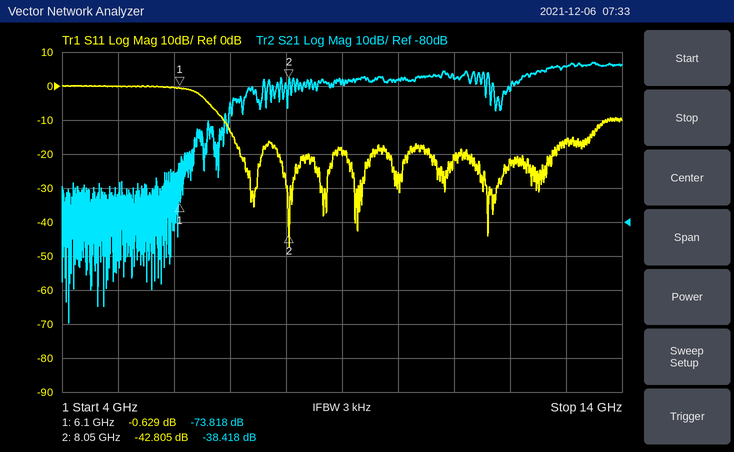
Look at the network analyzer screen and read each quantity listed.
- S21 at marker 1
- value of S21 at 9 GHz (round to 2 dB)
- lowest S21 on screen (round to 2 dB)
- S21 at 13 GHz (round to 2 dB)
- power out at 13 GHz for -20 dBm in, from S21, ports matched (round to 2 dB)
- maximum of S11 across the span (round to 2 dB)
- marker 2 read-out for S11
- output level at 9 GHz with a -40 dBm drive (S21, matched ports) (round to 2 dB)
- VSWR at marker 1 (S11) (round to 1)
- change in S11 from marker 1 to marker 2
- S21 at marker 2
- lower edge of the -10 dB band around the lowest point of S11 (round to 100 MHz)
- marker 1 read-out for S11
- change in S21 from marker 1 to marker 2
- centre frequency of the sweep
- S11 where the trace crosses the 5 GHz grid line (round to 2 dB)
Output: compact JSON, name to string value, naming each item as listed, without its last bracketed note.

{"S21 at marker 1": "-73.818 dB", "value of S21 at 9 GHz": "-38 dB", "lowest S21 on screen": "-110 dB", "S21 at 13 GHz": "-34 dB", "power out at 13 GHz for -20 dBm in, from S21, ports matched": "-54 dBm", "maximum of S11 across the span": "0 dB", "marker 2 read-out for S11": "-42.805 dB", "output level at 9 GHz with a -40 dBm drive (S21, matched ports)": "-78 dBm", "VSWR at marker 1 (S11)": "28", "change in S11 from marker 1 to marker 2": "-42.176 dB", "S21 at marker 2": "-38.418 dB", "lower edge of the -10 dB band around the lowest point of S11": "6.9 GHz", "marker 1 read-out for S11": "-0.629 dB", "change in S21 from marker 1 to marker 2": "35.400 dB", "centre frequency of the sweep": "9 GHz", "S11 where the trace crosses the 5 GHz grid line": "0 dB"}
